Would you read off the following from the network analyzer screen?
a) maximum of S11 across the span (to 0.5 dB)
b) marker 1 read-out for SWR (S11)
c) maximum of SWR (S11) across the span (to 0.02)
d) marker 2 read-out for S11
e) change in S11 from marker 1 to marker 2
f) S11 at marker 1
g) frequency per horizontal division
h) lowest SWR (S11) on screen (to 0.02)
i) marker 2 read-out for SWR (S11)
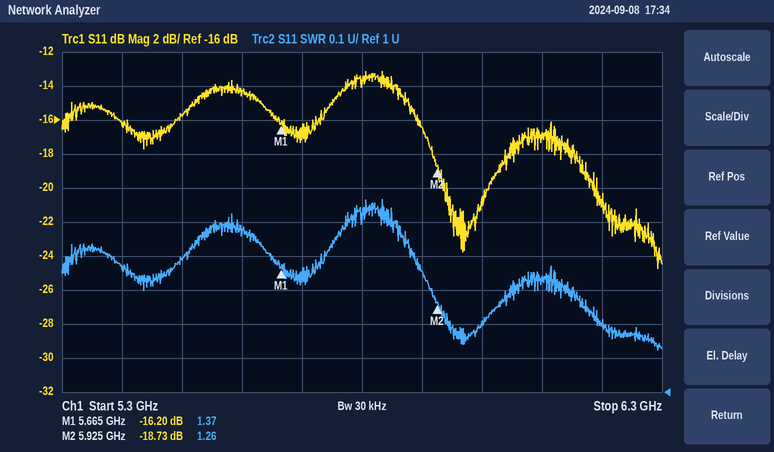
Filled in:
-13.0 dB
1.37
1.56
-18.73 dB
-2.53 dB
-16.20 dB
100 MHz
1.12
1.26
